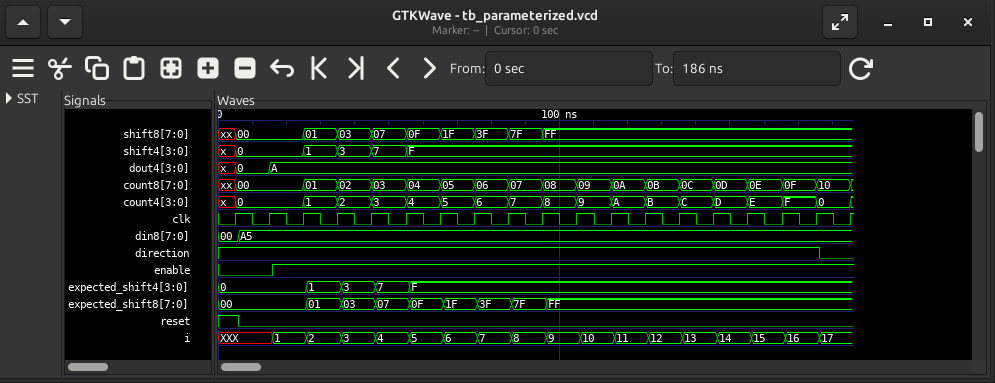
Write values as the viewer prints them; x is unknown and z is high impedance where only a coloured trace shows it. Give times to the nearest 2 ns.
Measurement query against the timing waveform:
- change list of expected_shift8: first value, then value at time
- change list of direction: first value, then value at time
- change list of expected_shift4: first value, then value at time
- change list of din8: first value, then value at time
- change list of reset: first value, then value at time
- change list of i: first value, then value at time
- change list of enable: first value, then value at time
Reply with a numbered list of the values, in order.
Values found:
1. 00, 01 at 26 ns, 03 at 36 ns, 07 at 46 ns, 0F at 56 ns, 1F at 66 ns, 3F at 76 ns, 7F at 86 ns, FF at 96 ns
2. 1, 0 at 176 ns
3. 0, 1 at 26 ns, 3 at 36 ns, 7 at 46 ns, F at 56 ns
4. 00, A5 at 6 ns
5. 1, 0 at 6 ns
6. XXX, 1 at 16 ns, 2 at 26 ns, 3 at 36 ns, 4 at 46 ns, 5 at 56 ns, 6 at 66 ns, 7 at 76 ns, 8 at 86 ns, 9 at 96 ns, 10 at 106 ns, 11 at 116 ns, 12 at 126 ns, 13 at 136 ns, 14 at 146 ns, 15 at 156 ns, 16 at 166 ns, 17 at 176 ns
7. 0, 1 at 16 ns
